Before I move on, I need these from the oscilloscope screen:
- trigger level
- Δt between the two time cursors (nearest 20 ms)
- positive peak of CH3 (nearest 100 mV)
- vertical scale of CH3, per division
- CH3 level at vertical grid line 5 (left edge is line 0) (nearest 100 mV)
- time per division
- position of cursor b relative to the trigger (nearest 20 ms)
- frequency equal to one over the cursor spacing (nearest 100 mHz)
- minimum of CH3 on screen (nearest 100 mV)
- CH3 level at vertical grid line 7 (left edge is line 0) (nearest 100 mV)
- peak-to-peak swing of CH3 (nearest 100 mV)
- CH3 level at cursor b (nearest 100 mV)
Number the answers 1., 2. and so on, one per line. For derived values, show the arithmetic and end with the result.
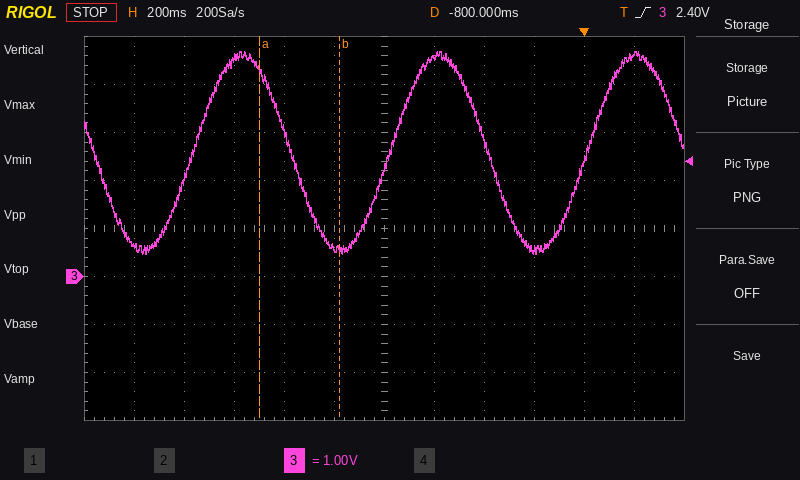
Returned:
1. 2.40 V
2. 320 ms
3. 4.7 V
4. 1 V
5. 600 mV
6. 200 ms
7. -980 ms
8. 1 / 320 ms ≈ 3.1 Hz
9. 500 mV
10. 4.6 V
11. 4.7 V − (500 mV) = 4.2 V
12. 600 mV
